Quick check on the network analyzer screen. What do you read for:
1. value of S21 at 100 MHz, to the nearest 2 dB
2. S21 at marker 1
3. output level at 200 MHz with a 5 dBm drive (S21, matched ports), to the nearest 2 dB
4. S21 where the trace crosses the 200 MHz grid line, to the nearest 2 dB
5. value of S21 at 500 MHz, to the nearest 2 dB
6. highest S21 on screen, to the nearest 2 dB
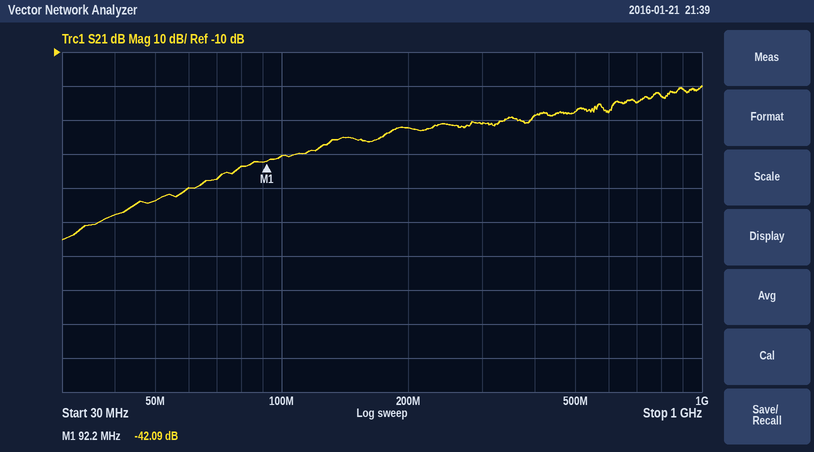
-40 dB
-42.09 dB
-28 dBm
-32 dB
-28 dB
-20 dB
